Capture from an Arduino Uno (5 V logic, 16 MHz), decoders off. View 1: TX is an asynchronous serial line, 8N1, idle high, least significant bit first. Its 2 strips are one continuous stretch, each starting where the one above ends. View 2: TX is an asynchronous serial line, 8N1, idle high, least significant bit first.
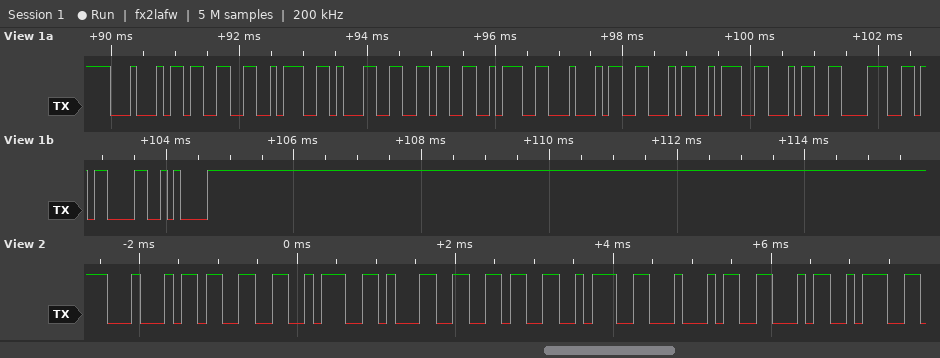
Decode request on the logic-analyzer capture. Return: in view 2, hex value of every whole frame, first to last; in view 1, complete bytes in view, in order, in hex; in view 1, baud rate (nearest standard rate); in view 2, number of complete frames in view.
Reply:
0x44 0x33 0x3A 0x31 0x36 0x3A 0x44 0x46 0x3A
44 33 3A 31 36 3A 44 46 3A 34 38 0D 0A
9600 baud
9
